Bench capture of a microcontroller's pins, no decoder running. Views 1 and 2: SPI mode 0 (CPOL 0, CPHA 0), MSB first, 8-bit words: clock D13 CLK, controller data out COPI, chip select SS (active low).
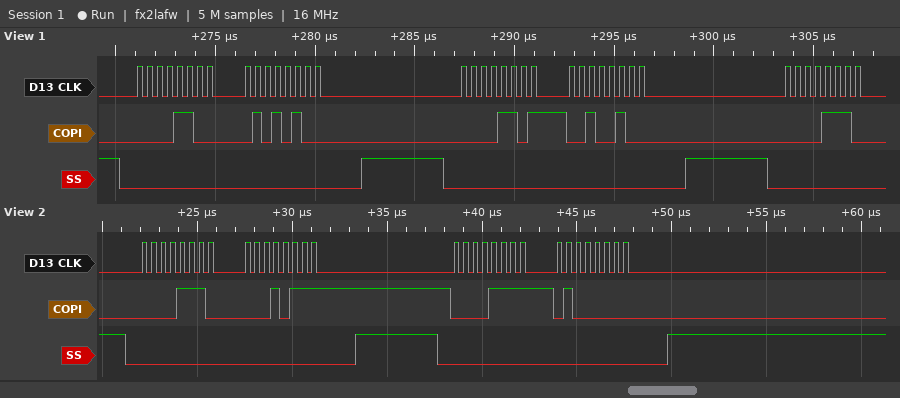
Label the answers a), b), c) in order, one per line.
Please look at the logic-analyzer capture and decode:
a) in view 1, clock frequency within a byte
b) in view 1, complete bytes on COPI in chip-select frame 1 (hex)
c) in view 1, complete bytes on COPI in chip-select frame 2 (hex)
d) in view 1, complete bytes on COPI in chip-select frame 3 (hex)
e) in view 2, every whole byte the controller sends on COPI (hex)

a) 2 MHz
b) 0x0C 0x54
c) 0x0D 0x24
d) 0x0E
e) 0E 17 0F 40
